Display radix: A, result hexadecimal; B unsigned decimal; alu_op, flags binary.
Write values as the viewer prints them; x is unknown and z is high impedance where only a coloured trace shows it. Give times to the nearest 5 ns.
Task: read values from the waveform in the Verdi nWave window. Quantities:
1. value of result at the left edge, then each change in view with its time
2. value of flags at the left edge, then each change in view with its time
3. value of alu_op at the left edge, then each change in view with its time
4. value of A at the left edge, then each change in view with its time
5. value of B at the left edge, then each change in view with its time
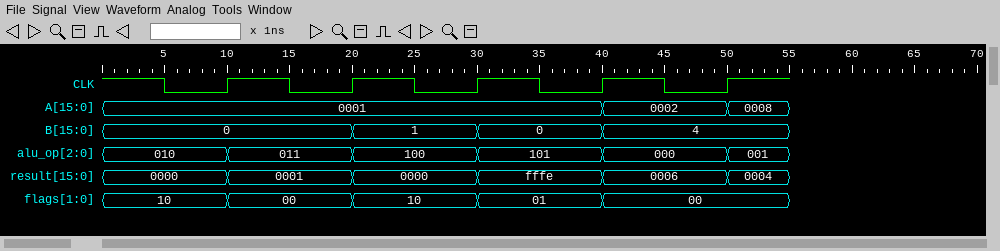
0000, 0001 at 10 ns, 0000 at 20 ns, fffe at 30 ns, 0006 at 40 ns, 0004 at 50 ns
10, 00 at 10 ns, 10 at 20 ns, 01 at 30 ns, 00 at 40 ns
010, 011 at 10 ns, 100 at 20 ns, 101 at 30 ns, 000 at 40 ns, 001 at 50 ns
0001, 0002 at 40 ns, 0008 at 50 ns
0, 1 at 20 ns, 0 at 30 ns, 4 at 40 ns
